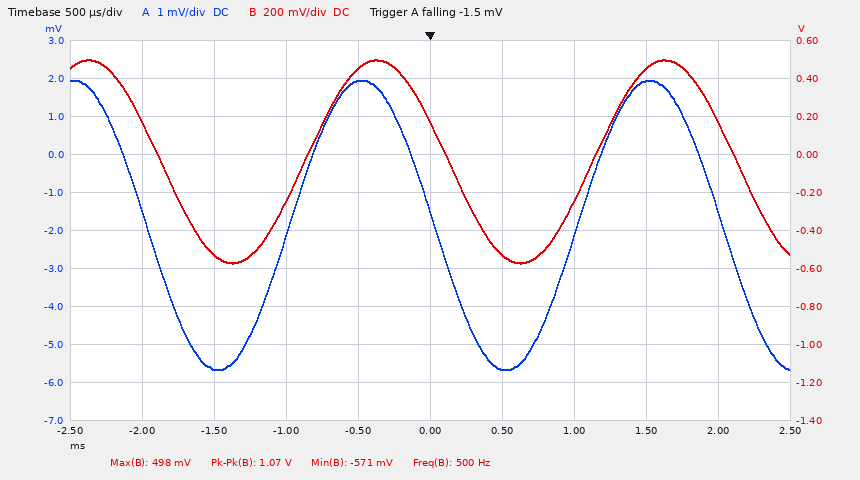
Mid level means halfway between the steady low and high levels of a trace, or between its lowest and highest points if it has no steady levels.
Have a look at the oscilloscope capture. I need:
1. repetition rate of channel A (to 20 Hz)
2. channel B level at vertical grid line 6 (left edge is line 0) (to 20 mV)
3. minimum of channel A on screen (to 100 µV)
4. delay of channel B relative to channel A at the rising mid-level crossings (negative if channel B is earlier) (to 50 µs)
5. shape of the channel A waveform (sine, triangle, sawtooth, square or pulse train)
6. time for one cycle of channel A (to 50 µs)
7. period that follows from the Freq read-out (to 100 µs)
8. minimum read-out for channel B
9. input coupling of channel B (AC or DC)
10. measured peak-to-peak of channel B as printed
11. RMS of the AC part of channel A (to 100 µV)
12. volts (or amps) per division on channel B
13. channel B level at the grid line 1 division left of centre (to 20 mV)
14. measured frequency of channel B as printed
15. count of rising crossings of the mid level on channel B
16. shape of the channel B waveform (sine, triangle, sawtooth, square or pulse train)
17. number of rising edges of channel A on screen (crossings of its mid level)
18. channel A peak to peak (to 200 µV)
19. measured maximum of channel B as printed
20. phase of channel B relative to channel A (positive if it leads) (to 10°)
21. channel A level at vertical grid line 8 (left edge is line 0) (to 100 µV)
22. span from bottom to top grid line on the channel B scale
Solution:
500 Hz
-520 mV
-5.7 mV
+100 µs
sine
2.00 ms
2.0 ms
-571 mV
DC
1.07 V
2.7 mV
200 mV
460 mV
500 Hz
2
sine
2
7.6 mV
498 mV
-20°
1.9 mV
2 V
